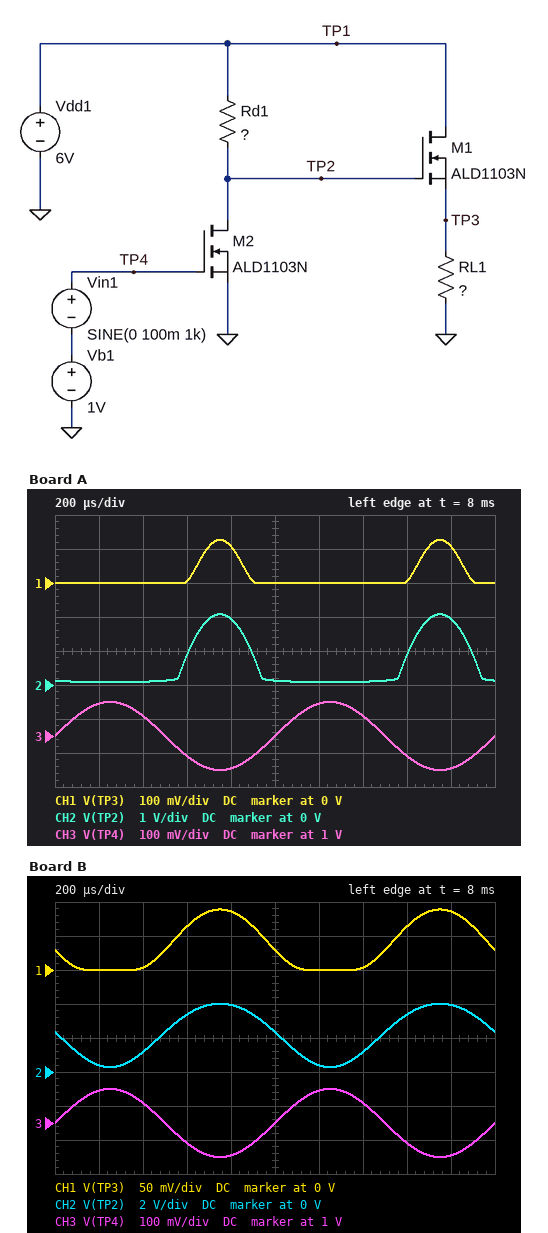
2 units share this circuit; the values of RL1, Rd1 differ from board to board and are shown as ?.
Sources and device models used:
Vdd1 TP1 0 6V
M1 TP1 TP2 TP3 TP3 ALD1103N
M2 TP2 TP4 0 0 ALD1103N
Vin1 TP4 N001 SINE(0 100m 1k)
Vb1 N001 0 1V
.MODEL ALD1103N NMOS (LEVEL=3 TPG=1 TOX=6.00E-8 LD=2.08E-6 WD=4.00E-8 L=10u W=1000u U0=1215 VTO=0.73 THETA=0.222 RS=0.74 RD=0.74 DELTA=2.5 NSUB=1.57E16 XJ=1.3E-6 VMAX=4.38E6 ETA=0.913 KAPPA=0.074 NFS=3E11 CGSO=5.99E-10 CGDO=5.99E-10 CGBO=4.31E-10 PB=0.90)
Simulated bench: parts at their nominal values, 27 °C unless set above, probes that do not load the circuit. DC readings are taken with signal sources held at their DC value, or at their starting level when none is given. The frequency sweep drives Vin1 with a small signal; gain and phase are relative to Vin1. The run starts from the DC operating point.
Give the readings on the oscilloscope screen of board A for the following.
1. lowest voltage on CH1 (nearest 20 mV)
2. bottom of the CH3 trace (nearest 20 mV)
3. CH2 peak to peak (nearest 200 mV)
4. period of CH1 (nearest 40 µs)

0 V
900 mV
2.0 V
1.00 ms
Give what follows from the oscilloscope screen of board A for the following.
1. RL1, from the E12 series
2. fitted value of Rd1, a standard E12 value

22 Ω
18 kΩ
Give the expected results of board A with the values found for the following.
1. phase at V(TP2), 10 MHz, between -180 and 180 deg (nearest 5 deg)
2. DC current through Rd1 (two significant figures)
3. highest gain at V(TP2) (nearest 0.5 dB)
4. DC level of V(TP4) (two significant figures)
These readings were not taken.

165 deg
330 µA
-1.5 dB
1.0 V
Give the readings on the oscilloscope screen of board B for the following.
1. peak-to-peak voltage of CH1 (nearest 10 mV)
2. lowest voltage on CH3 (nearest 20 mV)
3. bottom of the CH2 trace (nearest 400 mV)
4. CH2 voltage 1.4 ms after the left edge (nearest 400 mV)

90 mV
900 mV
400 mV
1.2 V
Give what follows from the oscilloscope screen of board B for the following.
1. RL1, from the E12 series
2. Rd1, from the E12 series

3.3 Ω
8.2 kΩ
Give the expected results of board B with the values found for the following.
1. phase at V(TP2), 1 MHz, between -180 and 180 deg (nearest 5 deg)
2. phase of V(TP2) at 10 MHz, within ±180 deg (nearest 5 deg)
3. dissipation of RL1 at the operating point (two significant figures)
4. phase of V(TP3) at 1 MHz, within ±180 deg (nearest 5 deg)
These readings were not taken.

170 deg
120 deg
260 µW
170 deg
